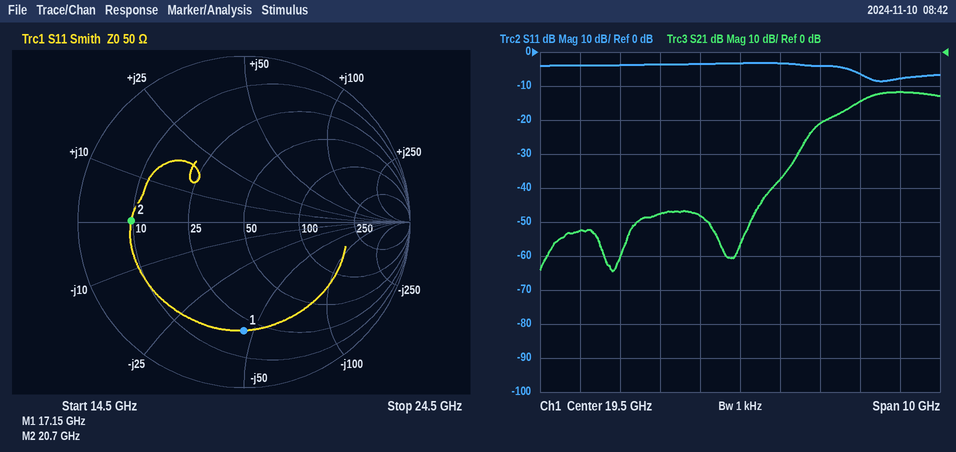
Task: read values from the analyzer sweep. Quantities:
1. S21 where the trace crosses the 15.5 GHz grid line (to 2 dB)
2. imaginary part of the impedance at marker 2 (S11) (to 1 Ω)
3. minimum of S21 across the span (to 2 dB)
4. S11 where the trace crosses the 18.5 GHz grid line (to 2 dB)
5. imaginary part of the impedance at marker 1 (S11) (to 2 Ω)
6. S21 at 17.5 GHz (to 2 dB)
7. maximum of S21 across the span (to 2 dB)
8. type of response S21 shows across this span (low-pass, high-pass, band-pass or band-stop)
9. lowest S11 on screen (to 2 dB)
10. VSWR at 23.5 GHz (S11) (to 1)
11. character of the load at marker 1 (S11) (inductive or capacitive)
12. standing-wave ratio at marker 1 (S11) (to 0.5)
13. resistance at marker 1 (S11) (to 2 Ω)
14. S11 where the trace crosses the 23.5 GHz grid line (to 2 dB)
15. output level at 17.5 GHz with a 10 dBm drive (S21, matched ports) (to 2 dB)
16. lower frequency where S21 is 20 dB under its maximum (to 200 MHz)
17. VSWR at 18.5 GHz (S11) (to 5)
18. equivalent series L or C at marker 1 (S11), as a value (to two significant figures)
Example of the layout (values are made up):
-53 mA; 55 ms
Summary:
-52 dB; 0 Ω; -64 dB; -4 dB; -46 Ω; -48 dB; -12 dB; high-pass; -8 dB; 2; capacitive; 5.0; 20 Ω; -8 dB; -38 dBm; 20.8 GHz; 5; 200 fF
